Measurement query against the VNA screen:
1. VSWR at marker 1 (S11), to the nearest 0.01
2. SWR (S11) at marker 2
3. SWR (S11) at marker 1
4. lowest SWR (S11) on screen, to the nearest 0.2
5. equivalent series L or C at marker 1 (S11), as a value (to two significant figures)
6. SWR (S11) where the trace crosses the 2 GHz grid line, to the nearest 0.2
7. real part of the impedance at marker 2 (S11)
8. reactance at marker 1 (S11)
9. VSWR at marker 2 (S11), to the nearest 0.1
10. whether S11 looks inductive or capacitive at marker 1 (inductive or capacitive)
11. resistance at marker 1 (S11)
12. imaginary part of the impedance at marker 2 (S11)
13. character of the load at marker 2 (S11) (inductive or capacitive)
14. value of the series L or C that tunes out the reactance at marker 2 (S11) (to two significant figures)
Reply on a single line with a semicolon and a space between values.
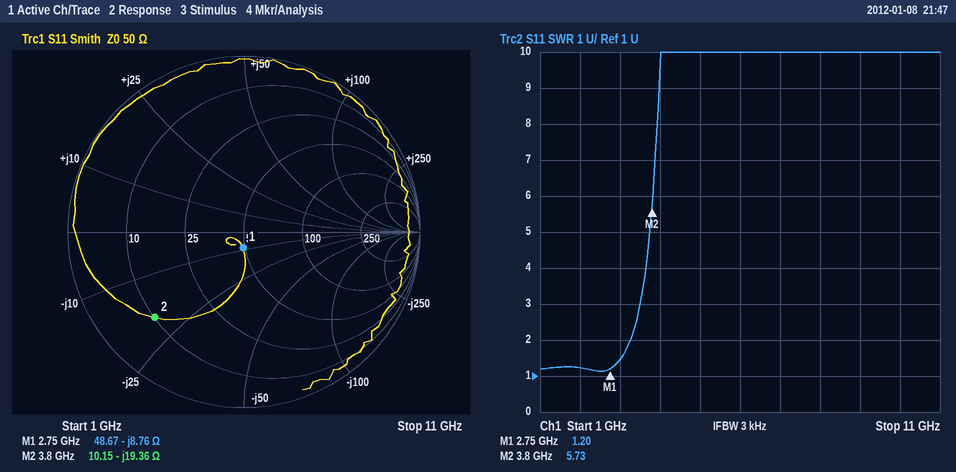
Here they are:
1.20; 5.73; 1.20; 1.2; 6.6 pF; 1.2; 10.15 Ω; -8.76 Ω; 5.7; capacitive; 48.67 Ω; -19.36 Ω; capacitive; 810 pH
